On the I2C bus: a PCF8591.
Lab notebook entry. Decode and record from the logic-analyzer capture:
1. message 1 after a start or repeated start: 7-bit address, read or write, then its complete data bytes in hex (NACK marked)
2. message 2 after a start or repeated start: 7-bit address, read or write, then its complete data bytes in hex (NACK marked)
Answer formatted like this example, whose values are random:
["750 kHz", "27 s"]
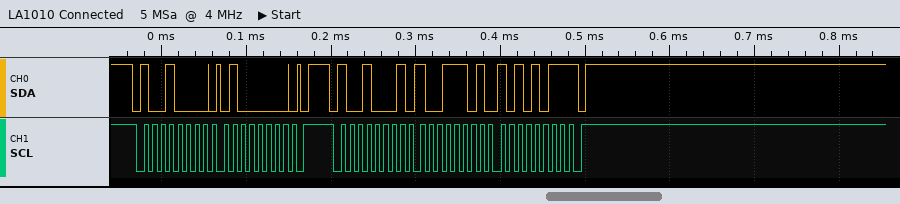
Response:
["0x48 write: 40", "0x48 read: 9D AB NACK"]
